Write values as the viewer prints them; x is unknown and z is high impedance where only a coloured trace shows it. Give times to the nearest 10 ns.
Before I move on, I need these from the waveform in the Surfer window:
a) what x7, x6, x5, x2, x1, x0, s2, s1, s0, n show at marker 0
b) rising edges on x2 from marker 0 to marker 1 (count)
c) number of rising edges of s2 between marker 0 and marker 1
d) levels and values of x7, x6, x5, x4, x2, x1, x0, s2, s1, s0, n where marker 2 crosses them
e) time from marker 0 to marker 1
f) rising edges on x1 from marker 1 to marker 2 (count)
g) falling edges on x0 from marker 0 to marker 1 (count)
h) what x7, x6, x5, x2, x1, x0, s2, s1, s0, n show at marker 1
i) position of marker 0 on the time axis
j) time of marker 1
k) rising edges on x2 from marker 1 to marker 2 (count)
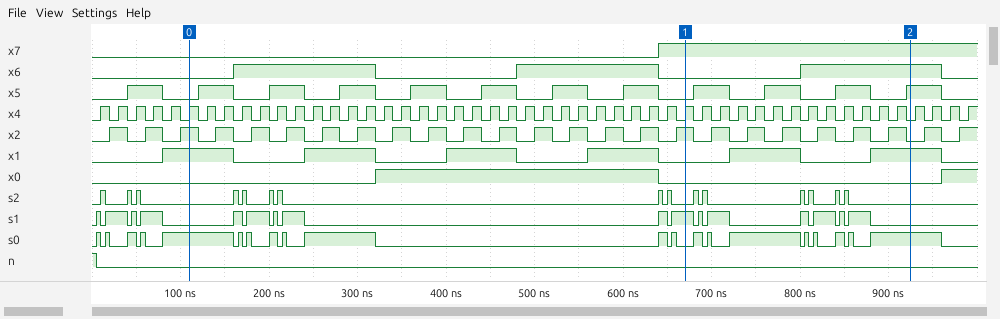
x7=0, x6=0, x5=0, x2=1, x1=1, x0=0, s2=0, s1=0, s0=1, n=0
14
6
x7=1, x6=1, x5=1, x4=0, x2=0, x1=1, x0=0, s2=0, s1=0, s0=1, n=0
560 ns
2
1
x7=1, x6=0, x5=0, x2=1, x1=0, x0=0, s2=0, s1=1, s0=0, n=0
110 ns
670 ns
6
